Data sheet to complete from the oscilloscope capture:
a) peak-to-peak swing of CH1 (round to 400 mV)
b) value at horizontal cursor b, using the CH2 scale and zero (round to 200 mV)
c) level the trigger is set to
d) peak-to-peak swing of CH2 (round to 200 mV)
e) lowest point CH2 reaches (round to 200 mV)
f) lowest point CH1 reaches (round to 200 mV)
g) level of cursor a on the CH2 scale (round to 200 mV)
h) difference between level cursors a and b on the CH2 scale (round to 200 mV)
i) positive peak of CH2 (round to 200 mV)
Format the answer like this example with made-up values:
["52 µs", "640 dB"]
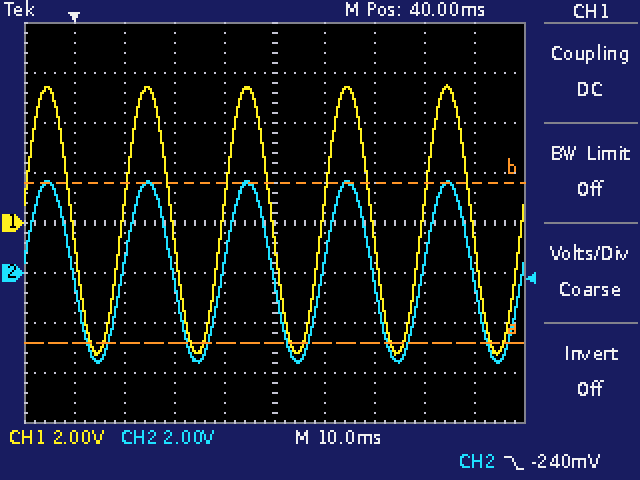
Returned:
["10.8 V", "3.6 V", "-240 mV", "7.2 V", "-3.6 V", "-5.2 V", "-2.8 V", "6.4 V", "3.6 V"]
